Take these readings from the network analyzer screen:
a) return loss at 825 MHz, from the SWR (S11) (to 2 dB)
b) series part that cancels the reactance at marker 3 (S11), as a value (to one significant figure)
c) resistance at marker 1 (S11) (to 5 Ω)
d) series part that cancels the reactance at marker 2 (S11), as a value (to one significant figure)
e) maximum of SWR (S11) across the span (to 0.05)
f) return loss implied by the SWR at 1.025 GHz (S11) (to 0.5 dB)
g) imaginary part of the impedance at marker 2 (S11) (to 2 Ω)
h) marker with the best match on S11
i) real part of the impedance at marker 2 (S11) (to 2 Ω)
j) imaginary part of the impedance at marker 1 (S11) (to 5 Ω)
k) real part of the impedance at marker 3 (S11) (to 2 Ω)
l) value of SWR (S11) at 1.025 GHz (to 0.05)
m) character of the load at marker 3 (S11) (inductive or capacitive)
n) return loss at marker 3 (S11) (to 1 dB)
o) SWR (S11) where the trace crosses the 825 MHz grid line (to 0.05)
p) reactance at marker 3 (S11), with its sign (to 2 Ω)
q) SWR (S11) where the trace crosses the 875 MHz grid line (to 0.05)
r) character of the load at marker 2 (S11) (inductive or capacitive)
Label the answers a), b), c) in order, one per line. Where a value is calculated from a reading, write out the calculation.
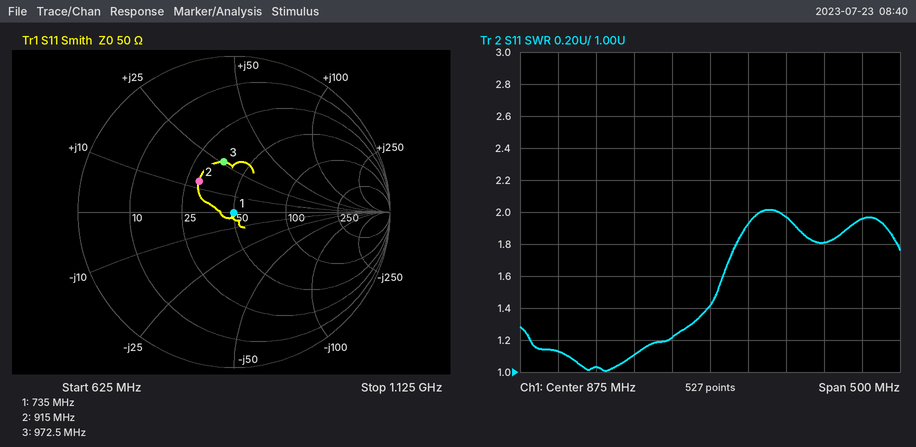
a) −20 log10((1.2 − 1)/(1.2 + 1)) ≈ 20.8 dB, so 20 dB to the nearest 2 dB
b) C = 1/(2π × 972.5 MHz × 26 Ω) ≈ 6 pF
c) 50 Ω
d) C = 1/(2π × 915 MHz × 12 Ω) ≈ 14.5 pF, so 10 pF to one significant figure
e) 2.00
f) −20 log10((1.8 − 1)/(1.8 + 1)) ≈ 10.9 dB, so 11.0 dB to the nearest 0.5 dB
g) +12 Ω
h) marker 1
i) 30 Ω
j) 0 Ω
k) 36 Ω
l) 1.80
m) inductive
n) 10 dB
o) 1.20
p) +26 Ω
q) 1.40
r) inductive
